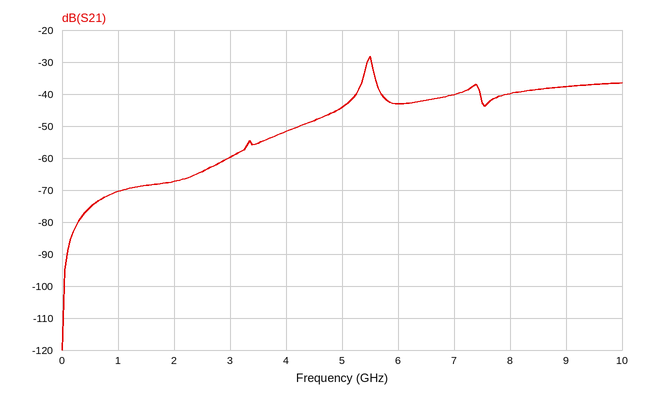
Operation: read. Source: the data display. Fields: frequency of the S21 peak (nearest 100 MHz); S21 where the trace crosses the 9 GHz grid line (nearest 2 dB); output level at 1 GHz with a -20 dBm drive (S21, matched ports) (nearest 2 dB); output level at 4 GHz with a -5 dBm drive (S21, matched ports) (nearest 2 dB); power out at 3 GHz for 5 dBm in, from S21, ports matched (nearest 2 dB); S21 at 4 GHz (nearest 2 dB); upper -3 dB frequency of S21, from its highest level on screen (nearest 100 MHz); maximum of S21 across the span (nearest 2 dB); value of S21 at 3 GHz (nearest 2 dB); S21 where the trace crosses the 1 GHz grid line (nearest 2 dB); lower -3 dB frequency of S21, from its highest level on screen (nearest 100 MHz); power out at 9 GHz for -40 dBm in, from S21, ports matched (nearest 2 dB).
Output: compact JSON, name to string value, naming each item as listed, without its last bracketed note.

{"frequency of the S21 peak": "5.5 GHz", "S21 where the trace crosses the 9 GHz grid line": "-38 dB", "output level at 1 GHz with a -20 dBm drive (S21, matched ports)": "-90 dBm", "output level at 4 GHz with a -5 dBm drive (S21, matched ports)": "-56 dBm", "power out at 3 GHz for 5 dBm in, from S21, ports matched": "-54 dBm", "S21 at 4 GHz": "-52 dB", "upper -3 dB frequency of S21, from its highest level on screen": "5.5 GHz", "maximum of S21 across the span": "-28 dB", "value of S21 at 3 GHz": "-60 dB", "S21 where the trace crosses the 1 GHz grid line": "-70 dB", "lower -3 dB frequency of S21, from its highest level on screen": "5.4 GHz", "power out at 9 GHz for -40 dBm in, from S21, ports matched": "-78 dBm"}
